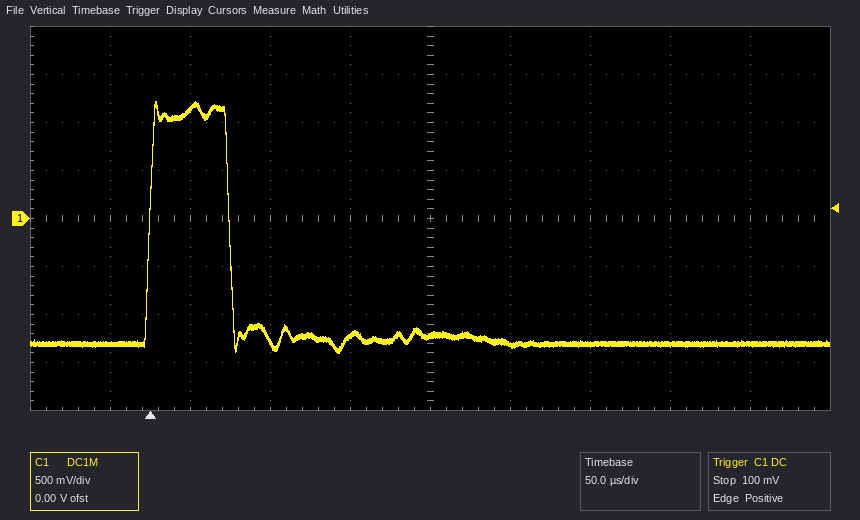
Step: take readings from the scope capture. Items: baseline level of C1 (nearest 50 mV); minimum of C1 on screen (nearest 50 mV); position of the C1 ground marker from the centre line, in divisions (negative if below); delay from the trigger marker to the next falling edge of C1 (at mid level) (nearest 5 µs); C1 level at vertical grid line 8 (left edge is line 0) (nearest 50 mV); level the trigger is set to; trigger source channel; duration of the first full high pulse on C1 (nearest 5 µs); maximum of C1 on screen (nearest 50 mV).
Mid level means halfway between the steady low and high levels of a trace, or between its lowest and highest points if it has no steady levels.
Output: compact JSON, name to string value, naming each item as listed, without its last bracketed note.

{"baseline level of C1": "-1.30 V", "minimum of C1 on screen": "-1.40 V", "position of the C1 ground marker from the centre line, in divisions": "0.0 div", "delay from the trigger marker to the next falling edge of C1 (at mid level)": "50 µs", "C1 level at vertical grid line 8 (left edge is line 0)": "-1.30 V", "level the trigger is set to": "100 mV", "trigger source channel": "C1", "duration of the first full high pulse on C1": "50 µs", "maximum of C1 on screen": "1.20 V"}
